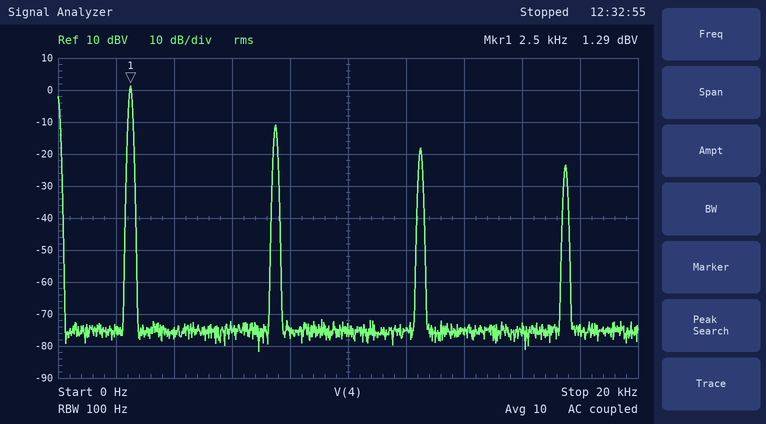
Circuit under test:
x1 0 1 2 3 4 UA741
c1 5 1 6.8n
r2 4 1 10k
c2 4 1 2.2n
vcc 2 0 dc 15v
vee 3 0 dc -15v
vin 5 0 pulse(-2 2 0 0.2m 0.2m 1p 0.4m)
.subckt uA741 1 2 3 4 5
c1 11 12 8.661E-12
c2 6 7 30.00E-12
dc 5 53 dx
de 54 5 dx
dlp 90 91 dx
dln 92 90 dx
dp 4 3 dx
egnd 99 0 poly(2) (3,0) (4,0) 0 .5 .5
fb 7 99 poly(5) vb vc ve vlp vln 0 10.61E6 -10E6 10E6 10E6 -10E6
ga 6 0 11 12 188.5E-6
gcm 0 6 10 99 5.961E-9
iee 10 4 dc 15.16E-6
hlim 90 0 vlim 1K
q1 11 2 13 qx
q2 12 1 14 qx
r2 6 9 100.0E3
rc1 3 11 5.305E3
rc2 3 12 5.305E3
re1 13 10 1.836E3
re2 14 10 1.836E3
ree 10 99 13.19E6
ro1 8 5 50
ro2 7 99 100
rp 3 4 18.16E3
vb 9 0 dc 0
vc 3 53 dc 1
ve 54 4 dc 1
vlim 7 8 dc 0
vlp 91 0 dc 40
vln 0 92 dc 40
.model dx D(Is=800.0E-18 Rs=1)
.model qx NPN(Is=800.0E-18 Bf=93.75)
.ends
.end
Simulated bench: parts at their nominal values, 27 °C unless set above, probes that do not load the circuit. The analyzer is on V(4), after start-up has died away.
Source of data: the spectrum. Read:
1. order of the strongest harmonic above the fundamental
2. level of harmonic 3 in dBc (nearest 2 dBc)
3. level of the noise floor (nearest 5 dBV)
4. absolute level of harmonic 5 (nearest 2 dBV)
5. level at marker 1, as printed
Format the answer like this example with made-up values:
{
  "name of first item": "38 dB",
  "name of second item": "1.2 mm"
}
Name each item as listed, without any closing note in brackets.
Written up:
{
  "order of the strongest harmonic above the fundamental": "3",
  "level of harmonic 3 in dBc": "-12 dBc",
  "level of the noise floor": "-75 dBV",
  "absolute level of harmonic 5": "-18 dBV",
  "level at marker 1, as printed": "1.29 dBV"
}
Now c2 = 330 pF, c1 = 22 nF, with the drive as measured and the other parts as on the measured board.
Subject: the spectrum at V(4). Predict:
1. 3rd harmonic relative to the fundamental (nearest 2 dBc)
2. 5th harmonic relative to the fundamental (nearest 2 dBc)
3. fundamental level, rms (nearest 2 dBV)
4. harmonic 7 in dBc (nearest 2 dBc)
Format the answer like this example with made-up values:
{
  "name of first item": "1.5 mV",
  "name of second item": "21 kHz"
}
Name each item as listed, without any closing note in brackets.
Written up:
{
  "3rd harmonic relative to the fundamental": "-8 dBc",
  "5th harmonic relative to the fundamental": "-10 dBc",
  "fundamental level, rms": "12 dBV",
  "harmonic 7 in dBc": "-12 dBc"
}
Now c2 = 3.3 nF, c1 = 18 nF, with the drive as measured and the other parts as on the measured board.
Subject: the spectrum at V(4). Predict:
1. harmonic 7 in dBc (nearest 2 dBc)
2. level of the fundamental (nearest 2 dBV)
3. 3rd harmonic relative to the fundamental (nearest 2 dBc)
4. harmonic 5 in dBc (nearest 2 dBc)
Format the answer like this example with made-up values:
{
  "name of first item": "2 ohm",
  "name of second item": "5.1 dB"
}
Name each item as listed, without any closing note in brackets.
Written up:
{
  "harmonic 7 in dBc": "-28 dBc",
  "level of the fundamental": "10 dBV",
  "3rd harmonic relative to the fundamental": "-14 dBc",
  "harmonic 5 in dBc": "-22 dBc"
}
